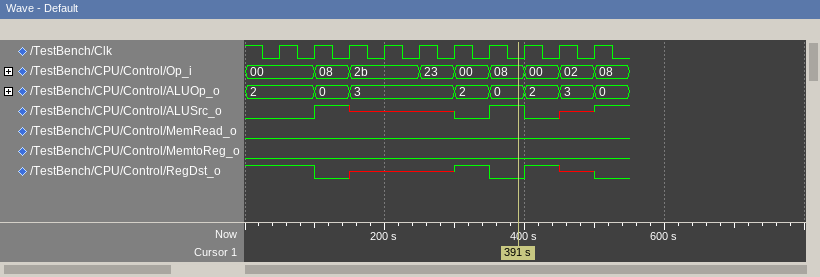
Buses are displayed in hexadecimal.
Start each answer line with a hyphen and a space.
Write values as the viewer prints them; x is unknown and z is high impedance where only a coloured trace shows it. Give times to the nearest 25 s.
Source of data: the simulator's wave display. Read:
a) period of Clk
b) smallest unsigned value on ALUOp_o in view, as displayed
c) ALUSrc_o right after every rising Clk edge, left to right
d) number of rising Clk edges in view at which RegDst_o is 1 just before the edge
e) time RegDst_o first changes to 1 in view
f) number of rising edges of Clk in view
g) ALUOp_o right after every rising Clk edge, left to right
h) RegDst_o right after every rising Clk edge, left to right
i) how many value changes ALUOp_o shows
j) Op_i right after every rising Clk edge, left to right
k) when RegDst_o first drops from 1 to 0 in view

- 50 s
- 0
- 0 1 x x x 0 1 0 x 1
- 4
- 300 s
- 10
- 2, 0, 3, 3, 3, 2, 0, 2, 3, 0
- 1 0 x x x 1 0 1 x 0
- 7
- 00, 08, 2b, 2b, 23, 00, 08, 00, 02, 08
- 100 s
